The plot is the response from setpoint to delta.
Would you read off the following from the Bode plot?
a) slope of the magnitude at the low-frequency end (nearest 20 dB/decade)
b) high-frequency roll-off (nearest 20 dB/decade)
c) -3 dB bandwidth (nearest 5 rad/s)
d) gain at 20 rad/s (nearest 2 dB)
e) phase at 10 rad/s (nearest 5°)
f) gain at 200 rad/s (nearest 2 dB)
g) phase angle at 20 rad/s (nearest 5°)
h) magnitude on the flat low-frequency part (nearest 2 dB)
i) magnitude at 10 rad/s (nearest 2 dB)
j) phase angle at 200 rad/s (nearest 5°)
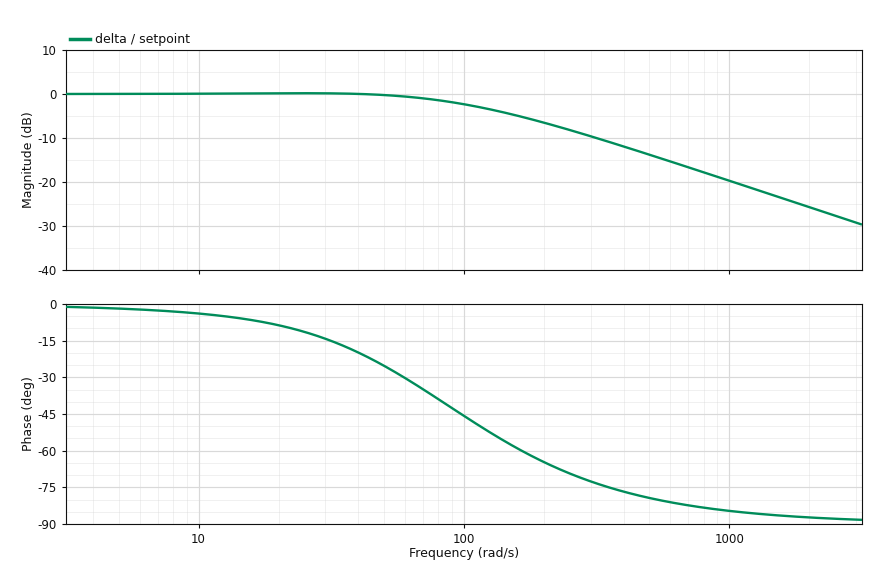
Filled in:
0 dB/decade
-20 dB/decade
115 rad/s
0 dB
-5°
-6 dB
-10°
0 dB
0 dB
-65°
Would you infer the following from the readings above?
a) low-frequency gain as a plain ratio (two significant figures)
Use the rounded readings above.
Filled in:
1.0
